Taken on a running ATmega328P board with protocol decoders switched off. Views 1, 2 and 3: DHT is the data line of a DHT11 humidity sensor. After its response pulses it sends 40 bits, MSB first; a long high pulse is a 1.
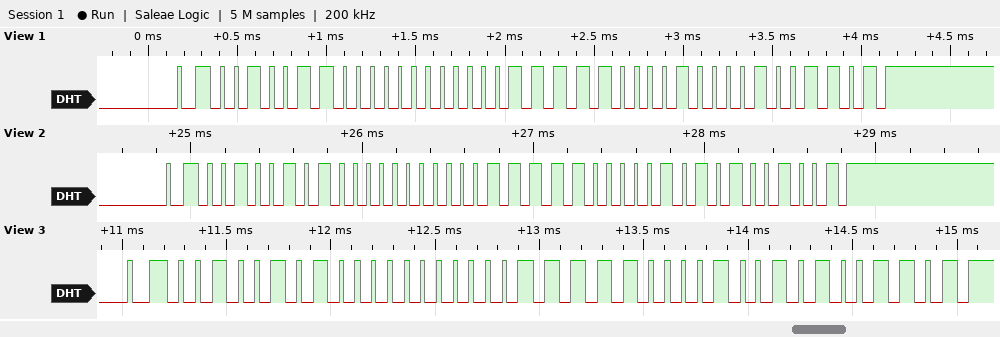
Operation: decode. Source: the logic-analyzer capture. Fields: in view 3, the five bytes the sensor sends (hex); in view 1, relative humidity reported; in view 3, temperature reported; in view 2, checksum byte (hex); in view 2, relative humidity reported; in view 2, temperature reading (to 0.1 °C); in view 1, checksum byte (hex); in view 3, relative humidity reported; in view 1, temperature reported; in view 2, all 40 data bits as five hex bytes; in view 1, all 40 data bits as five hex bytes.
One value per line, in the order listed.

25 00 1F 09 4D
38 %
31.9 °C
0x49
37 %
31.5 °C
0x4D
37 %
31.8 °C
25 00 1F 05 49
26 00 1F 08 4D
